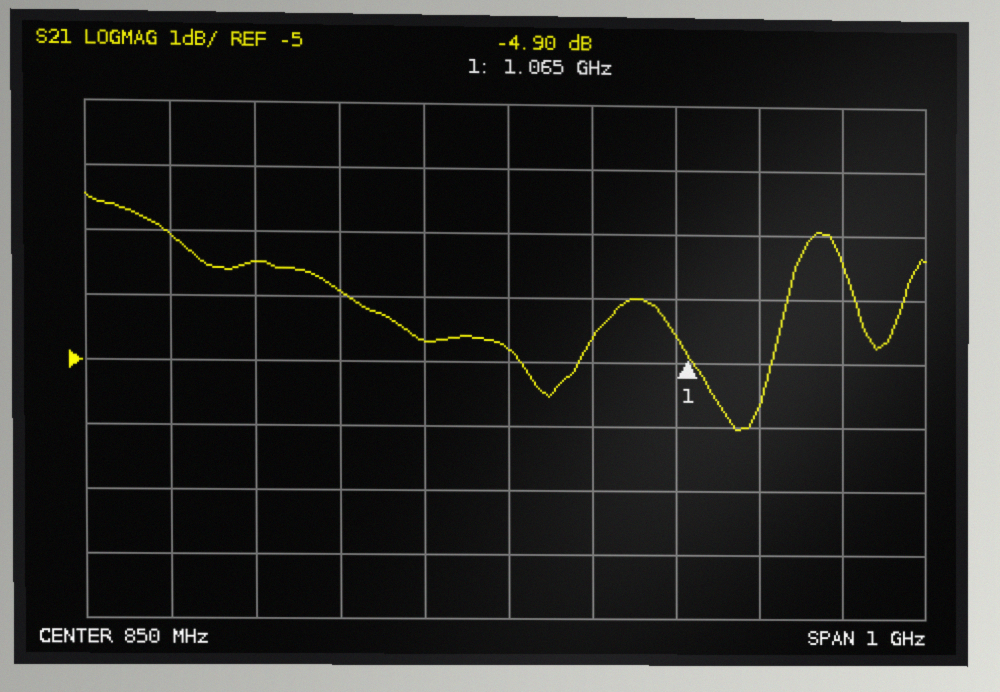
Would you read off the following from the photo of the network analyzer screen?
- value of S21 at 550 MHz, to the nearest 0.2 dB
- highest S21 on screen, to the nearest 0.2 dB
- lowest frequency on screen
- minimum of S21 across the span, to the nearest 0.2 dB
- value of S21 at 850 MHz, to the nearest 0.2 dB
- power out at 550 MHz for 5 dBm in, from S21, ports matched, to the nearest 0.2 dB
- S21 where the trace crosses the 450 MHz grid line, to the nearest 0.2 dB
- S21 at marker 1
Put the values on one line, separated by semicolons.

-3.4 dB; -2.4 dB; 350 MHz; -6.0 dB; -4.8 dB; 1.6 dBm; -3.0 dB; -4.90 dB
